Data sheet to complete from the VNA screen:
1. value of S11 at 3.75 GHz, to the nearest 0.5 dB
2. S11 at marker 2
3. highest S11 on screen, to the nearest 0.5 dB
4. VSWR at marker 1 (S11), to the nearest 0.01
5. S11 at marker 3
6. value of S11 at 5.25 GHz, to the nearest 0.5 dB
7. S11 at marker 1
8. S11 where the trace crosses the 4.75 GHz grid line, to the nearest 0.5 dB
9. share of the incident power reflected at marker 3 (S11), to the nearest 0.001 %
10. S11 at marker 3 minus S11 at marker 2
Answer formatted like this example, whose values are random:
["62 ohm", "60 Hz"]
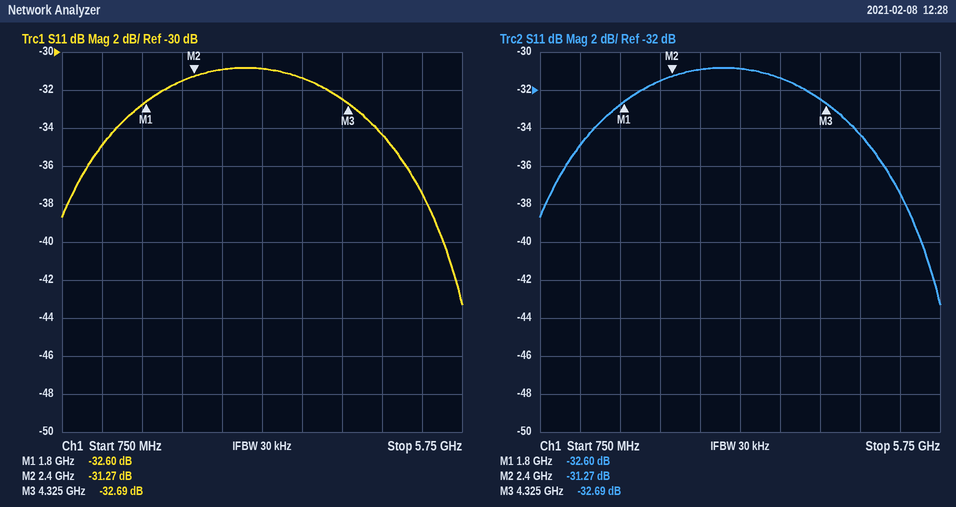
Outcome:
["-31.5 dB", "-31.27 dB", "-31.0 dB", "1.05", "-32.69 dB", "-37.5 dB", "-32.60 dB", "-34.5 dB", "0.054 %", "-1.42 dB"]
